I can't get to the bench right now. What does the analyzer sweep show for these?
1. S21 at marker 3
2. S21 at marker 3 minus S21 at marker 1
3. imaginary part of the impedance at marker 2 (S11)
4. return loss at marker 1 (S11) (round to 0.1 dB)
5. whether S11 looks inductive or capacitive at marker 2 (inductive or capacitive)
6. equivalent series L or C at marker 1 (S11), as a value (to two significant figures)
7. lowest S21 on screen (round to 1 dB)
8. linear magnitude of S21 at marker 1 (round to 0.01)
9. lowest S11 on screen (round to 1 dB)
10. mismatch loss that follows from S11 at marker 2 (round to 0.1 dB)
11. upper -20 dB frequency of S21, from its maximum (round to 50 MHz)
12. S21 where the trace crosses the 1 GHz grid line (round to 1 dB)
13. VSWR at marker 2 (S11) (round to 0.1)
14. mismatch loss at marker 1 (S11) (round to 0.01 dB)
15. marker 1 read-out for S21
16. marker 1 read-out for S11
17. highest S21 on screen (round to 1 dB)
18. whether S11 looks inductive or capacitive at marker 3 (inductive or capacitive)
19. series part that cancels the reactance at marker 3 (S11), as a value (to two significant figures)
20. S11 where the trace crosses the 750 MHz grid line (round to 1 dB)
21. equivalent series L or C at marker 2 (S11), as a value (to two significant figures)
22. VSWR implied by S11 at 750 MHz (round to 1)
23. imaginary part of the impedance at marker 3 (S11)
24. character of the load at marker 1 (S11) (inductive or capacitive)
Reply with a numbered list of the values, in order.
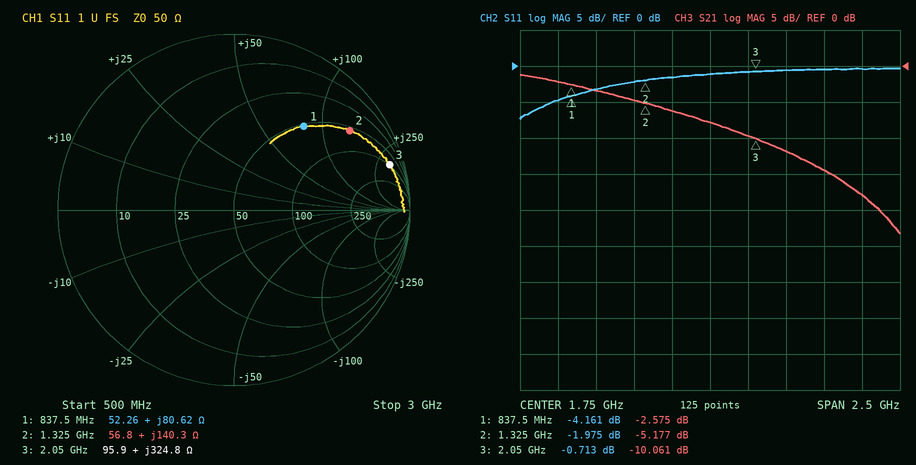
1. -10.061 dB
2. -7.486 dB
3. +140.3 Ω
4. 4.2 dB
5. inductive
6. 15 nH
7. -23 dB
8. 0.74
9. -7 dB
10. 4.4 dB
11. 2.90 GHz
12. -3 dB
13. 8.8
14. 2.10 dB
15. -2.575 dB
16. -4.161 dB
17. -1 dB
18. inductive
19. 240 fF
20. -5 dB
21. 17 nH
22. 4
23. +324.8 Ω
24. inductive
